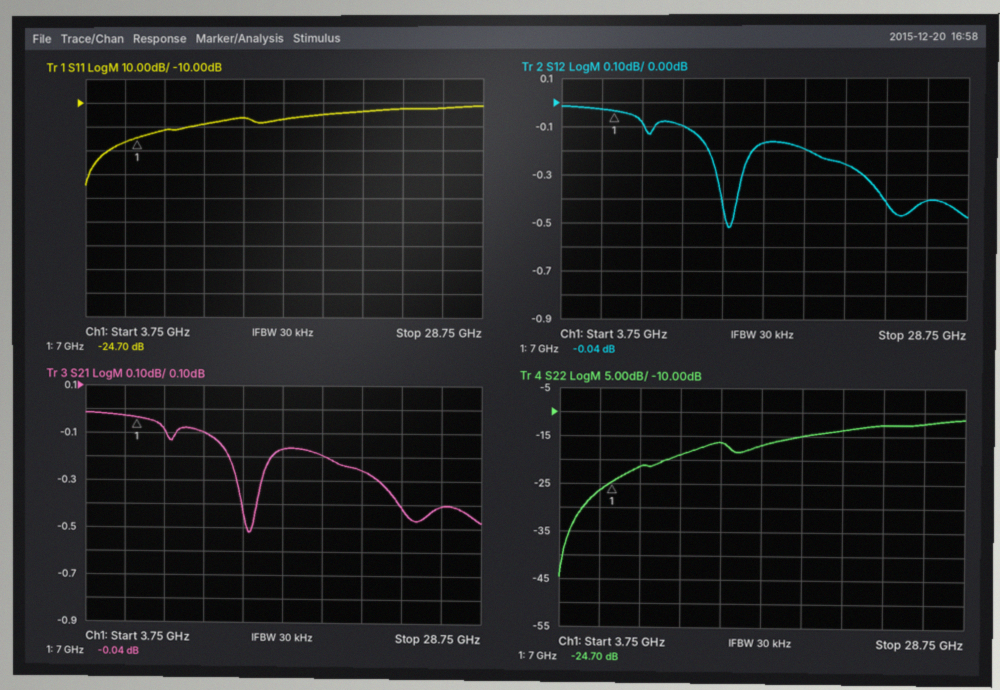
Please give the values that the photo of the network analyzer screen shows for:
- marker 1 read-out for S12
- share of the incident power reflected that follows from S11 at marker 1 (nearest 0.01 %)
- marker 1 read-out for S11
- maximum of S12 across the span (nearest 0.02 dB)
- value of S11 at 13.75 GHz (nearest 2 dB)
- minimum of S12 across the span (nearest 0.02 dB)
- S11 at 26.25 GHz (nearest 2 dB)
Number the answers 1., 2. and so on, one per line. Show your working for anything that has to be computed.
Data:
1. -0.04 dB
2. 10^(-24.7/10) ≈ 0.34 %
3. -24.70 dB
4. -0.02 dB
5. -16 dB
6. -0.52 dB
7. -12 dB
